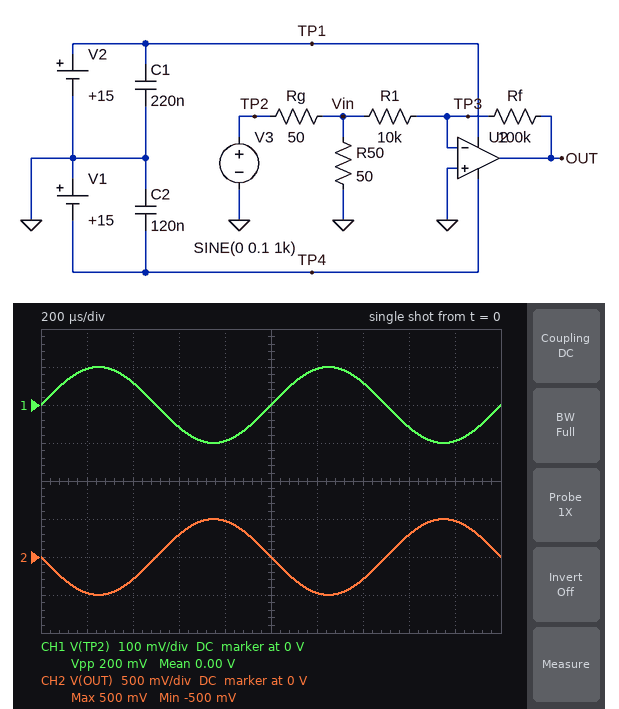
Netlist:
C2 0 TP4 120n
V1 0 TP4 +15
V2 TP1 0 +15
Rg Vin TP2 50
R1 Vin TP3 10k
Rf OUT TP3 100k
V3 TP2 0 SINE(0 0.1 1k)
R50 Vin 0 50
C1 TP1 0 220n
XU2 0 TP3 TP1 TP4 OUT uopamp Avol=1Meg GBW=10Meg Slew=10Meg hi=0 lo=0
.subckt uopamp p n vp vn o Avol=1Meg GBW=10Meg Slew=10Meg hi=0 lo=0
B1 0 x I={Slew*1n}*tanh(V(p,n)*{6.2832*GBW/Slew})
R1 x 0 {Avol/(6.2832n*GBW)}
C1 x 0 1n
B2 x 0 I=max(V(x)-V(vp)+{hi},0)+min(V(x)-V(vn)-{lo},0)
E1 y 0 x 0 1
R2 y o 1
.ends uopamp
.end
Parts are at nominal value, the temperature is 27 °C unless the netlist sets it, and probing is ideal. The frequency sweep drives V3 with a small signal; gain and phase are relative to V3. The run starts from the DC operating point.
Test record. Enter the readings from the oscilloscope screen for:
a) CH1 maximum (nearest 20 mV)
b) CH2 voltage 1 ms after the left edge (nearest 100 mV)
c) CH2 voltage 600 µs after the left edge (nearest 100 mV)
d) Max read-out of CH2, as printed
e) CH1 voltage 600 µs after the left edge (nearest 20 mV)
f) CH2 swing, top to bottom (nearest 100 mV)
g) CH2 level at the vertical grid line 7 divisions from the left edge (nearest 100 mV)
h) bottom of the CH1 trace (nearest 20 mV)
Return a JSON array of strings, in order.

["100 mV", "0 V", "300 mV", "500 mV", "-60 mV", "1.0 V", "-300 mV", "-100 mV"]
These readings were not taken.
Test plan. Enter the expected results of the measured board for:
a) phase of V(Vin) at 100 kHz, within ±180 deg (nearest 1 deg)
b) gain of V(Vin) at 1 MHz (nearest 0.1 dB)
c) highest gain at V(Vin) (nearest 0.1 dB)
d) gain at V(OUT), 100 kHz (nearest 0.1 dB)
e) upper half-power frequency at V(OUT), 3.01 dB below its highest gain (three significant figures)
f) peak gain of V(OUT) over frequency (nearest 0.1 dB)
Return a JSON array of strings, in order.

["0 deg", "-6.0 dB", "-6.0 dB", "13.9 dB", "911 kHz", "14.0 dB"]
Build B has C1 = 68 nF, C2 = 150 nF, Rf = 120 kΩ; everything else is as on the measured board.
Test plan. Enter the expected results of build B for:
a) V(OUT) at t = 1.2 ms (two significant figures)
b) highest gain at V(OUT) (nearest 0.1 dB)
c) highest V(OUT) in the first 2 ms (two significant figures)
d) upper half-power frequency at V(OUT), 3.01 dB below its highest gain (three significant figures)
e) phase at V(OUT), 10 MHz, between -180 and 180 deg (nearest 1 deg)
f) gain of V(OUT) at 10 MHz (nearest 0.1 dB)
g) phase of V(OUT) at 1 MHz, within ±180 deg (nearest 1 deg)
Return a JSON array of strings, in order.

["-570 mV", "15.5 dB", "600 mV", "771 kHz", "94 deg", "-6.7 dB", "128 deg"]
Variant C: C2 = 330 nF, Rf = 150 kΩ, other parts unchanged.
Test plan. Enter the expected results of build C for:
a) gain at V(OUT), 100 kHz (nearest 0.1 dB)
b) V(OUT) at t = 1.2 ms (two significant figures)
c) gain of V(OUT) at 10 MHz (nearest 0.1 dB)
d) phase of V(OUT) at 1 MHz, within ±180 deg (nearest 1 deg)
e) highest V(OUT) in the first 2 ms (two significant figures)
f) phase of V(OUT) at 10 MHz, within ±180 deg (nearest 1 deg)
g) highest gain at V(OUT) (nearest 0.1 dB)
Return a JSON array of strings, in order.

["17.4 dB", "-710 mV", "-6.6 dB", "122 deg", "750 mV", "94 deg", "17.5 dB"]
